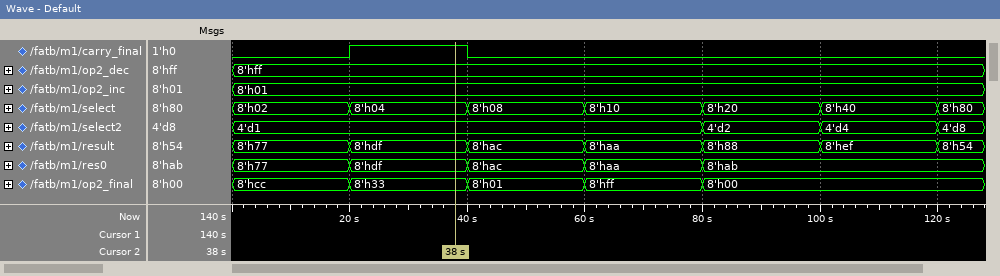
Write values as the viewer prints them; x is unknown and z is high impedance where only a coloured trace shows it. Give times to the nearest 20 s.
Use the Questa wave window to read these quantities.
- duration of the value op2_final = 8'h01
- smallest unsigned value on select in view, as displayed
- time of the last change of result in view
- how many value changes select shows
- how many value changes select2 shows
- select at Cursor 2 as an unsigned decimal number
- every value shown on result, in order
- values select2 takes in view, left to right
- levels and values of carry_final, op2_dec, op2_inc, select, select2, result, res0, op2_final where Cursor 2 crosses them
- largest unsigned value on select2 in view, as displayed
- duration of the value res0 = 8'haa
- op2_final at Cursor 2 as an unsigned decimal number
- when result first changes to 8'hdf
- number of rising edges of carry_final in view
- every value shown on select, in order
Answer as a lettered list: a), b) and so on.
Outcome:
a) 20 s
b) 8'h02
c) 120 s
d) 6
e) 3
f) 4
g) 8'h77, 8'hdf, 8'hac, 8'haa, 8'h88, 8'hef, 8'h54
h) 4'd1, 4'd2, 4'd4, 4'd8
i) carry_final=1, op2_dec=8'hff, op2_inc=8'h01, select=8'h04, select2=4'd1, result=8'hdf, res0=8'hdf, op2_final=8'h33
j) 4'd8
k) 20 s
l) 51
m) 20 s
n) 1
o) 8'h02, 8'h04, 8'h08, 8'h10, 8'h20, 8'h40, 8'h80
